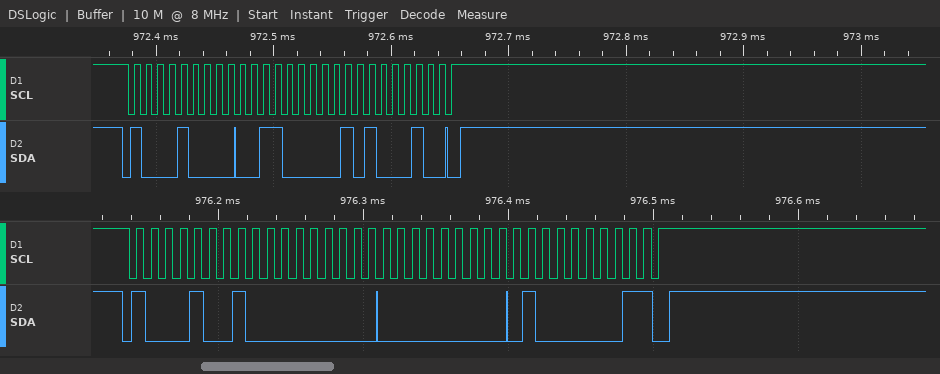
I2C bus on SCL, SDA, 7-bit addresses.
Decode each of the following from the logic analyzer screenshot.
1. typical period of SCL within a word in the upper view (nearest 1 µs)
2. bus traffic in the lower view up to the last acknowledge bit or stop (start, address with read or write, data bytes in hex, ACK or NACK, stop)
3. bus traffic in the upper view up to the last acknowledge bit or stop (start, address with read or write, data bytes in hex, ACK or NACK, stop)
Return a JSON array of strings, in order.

["10 µs", "start, address 44 read ACK, 00 ACK, 00 ACK, 81 NACK, stop", "start, address 44 write ACK, 30 ACK, A2 ACK, stop"]
